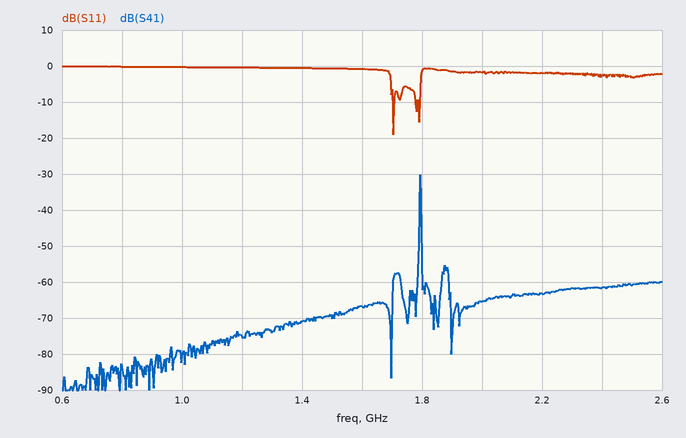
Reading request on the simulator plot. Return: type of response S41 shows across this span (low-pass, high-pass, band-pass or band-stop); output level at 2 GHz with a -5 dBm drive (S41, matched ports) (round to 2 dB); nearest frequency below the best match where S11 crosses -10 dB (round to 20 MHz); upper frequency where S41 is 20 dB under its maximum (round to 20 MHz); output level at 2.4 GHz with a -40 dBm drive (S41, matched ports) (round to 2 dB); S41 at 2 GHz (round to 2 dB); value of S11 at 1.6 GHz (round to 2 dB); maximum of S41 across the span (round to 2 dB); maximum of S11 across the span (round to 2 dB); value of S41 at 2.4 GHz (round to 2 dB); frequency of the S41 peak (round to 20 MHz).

band-pass
-70 dBm
1.70 GHz
1.80 GHz
-102 dBm
-66 dB
0 dB
-30 dB
0 dB
-62 dB
1.80 GHz
